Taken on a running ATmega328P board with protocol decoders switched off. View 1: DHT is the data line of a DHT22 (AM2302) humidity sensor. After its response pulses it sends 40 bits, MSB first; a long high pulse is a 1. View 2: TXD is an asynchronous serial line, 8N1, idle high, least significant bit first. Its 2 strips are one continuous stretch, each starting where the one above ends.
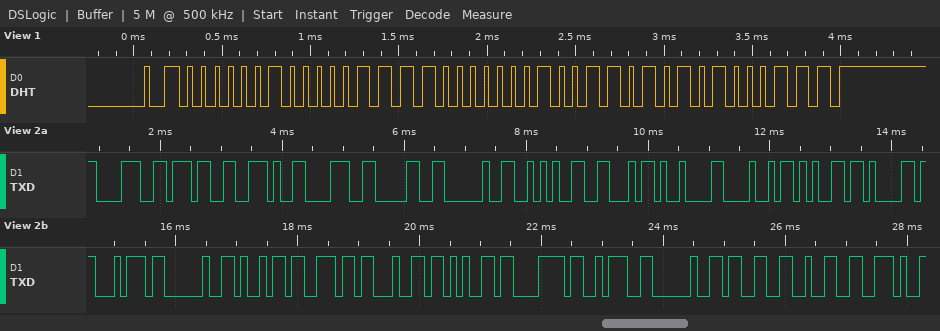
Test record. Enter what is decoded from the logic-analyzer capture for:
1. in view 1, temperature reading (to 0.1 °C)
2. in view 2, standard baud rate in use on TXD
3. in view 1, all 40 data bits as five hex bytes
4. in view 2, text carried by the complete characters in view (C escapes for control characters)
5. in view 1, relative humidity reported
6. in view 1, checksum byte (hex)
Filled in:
30.9 °C
9600 baud
02 0F 01 35 47
"87.80 *F\tHeat index: 32."
52.7 %
0x47
